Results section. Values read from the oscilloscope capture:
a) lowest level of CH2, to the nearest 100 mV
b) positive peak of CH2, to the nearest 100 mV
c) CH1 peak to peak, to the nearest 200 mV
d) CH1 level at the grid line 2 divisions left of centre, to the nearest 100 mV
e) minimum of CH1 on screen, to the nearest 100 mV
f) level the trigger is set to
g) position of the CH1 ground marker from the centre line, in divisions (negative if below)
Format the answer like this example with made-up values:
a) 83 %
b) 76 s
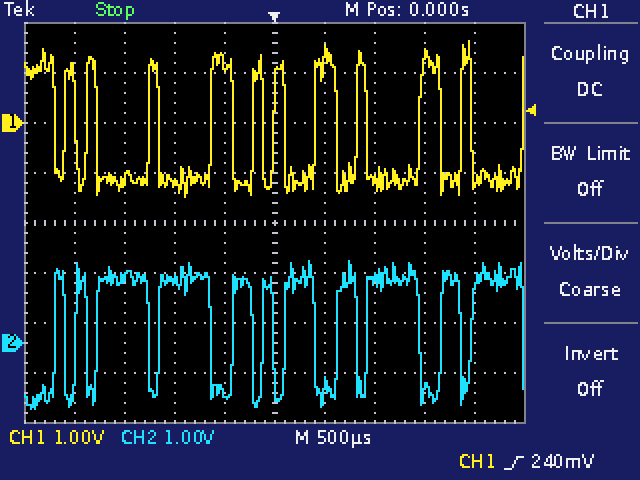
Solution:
a) -1.3 V
b) 1.6 V
c) 3.2 V
d) -1.2 V
e) -1.5 V
f) 240 mV
g) +2.0 div
